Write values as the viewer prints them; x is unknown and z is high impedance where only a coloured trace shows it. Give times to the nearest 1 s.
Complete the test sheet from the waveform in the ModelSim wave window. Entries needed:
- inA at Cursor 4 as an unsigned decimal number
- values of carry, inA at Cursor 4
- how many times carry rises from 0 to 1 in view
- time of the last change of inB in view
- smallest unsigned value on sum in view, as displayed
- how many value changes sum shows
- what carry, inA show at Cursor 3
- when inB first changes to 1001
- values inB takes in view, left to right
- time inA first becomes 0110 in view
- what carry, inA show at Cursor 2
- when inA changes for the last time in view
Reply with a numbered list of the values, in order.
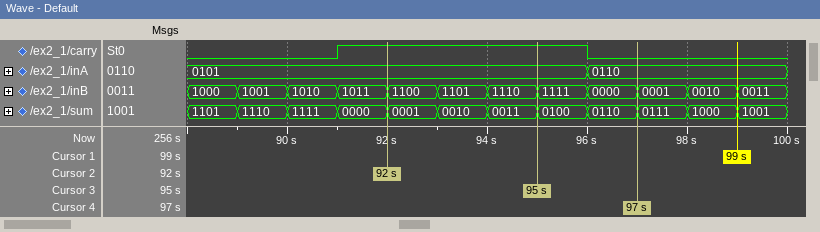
1. 6
2. carry=0, inA=0110
3. 1
4. 99 s
5. 0000
6. 11
7. carry=1, inA=0101
8. 89 s
9. 1000, 1001, 1010, 1011, 1100, 1101, 1110, 1111, 0000, 0001, 0010, 0011
10. 96 s
11. carry=1, inA=0101
12. 96 s
